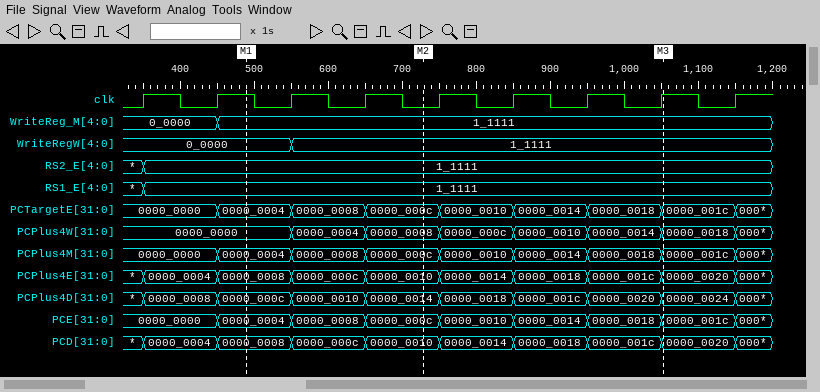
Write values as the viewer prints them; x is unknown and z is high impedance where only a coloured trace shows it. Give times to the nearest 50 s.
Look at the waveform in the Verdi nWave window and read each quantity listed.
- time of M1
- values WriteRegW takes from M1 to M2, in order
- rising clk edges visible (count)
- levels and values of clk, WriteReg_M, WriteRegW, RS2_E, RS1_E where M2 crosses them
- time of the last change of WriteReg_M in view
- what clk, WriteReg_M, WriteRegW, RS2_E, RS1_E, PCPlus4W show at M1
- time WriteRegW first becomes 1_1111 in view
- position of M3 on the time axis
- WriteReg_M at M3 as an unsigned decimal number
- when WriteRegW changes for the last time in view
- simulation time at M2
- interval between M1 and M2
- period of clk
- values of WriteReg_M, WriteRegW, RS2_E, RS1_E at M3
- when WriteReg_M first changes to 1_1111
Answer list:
500 s
0_0000, 1_1111
9
clk=0, WriteReg_M=1_1111, WriteRegW=1_1111, RS2_E=1_1111, RS1_E=1_1111
450 s
clk=1, WriteReg_M=1_1111, WriteRegW=0_0000, RS2_E=1_1111, RS1_E=1_1111, PCPlus4W=0000_0000
550 s
1050 s
31
550 s
750 s
250 s
100 s
WriteReg_M=1_1111, WriteRegW=1_1111, RS2_E=1_1111, RS1_E=1_1111
450 s
